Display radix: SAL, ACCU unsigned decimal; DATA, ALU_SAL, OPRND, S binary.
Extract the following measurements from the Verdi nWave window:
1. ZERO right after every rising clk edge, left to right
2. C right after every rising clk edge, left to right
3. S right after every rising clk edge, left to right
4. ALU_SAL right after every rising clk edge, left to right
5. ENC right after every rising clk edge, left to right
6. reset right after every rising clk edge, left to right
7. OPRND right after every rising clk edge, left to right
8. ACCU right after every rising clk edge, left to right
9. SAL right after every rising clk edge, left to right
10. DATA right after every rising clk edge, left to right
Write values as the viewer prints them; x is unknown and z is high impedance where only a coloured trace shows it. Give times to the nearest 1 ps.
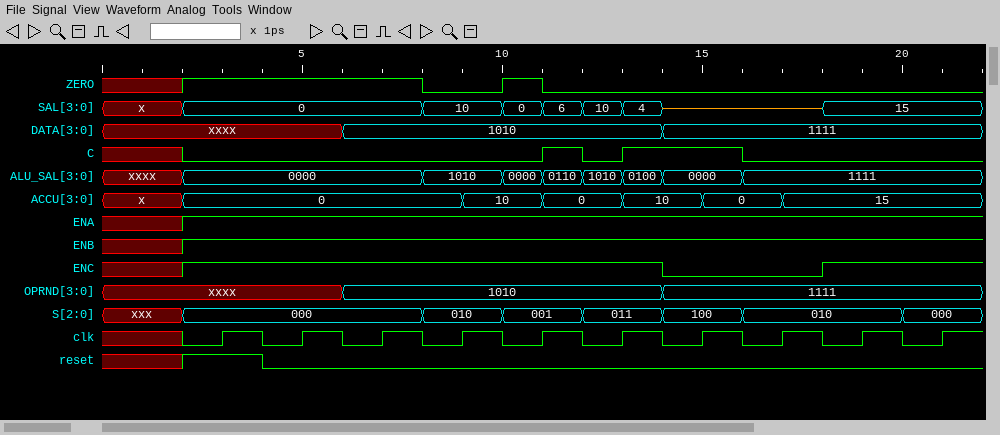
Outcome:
1 1 1 0 0 0 0 0 0 0
0 0 0 0 1 1 1 0 0 0
000, 000, 000, 010, 001, 011, 100, 010, 010, 000
0000, 0000, 0000, 1010, 0110, 0100, 0000, 1111, 1111, 1111
1 1 1 1 1 1 0 0 1 1
1 0 0 0 0 0 0 0 0 0
xxxx, xxxx, 1010, 1010, 1010, 1010, 1111, 1111, 1111, 1111
0, 0, 0, 10, 0, 10, 0, 15, 15, 15
0, 0, 0, 10, 6, 4, z, z, 15, 15
xxxx, xxxx, 1010, 1010, 1010, 1010, 1111, 1111, 1111, 1111
